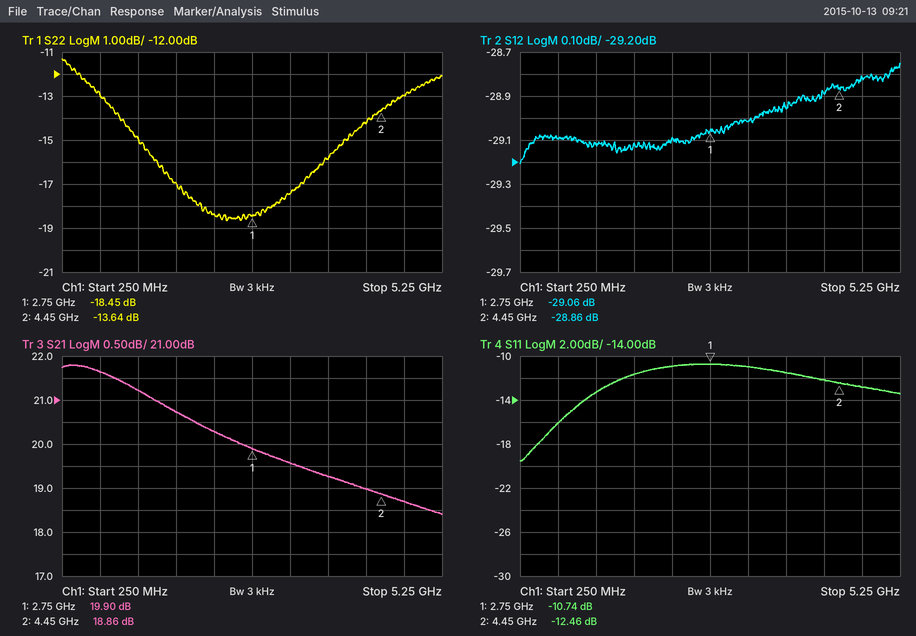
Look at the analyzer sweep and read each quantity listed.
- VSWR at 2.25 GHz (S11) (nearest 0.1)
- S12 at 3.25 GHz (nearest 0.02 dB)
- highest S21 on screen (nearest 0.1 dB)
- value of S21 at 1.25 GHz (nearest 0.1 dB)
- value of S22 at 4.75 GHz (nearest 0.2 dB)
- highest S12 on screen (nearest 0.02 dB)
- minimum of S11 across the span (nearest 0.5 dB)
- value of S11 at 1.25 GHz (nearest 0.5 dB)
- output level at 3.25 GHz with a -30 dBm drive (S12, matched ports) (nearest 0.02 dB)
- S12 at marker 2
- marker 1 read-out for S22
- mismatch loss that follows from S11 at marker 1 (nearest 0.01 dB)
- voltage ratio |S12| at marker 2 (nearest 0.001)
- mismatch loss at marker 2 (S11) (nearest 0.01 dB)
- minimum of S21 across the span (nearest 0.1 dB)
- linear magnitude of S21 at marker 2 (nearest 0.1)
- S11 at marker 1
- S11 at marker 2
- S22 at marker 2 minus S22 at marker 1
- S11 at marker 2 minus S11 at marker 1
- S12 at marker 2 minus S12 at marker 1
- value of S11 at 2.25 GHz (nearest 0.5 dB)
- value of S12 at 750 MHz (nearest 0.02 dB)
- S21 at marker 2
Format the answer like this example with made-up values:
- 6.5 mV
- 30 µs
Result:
- 1.8
- -29.02 dB
- 21.8 dB
- 21.2 dB
- -13.0 dB
- -28.76 dB
- -19.5 dB
- -13.5 dB
- -59.02 dBm
- -28.86 dB
- -18.45 dB
- 0.38 dB
- 0.036
- 0.25 dB
- 18.4 dB
- 8.8
- -10.74 dB
- -12.46 dB
- 4.81 dB
- -1.72 dB
- 0.20 dB
- -11.0 dB
- -29.10 dB
- 18.86 dB
